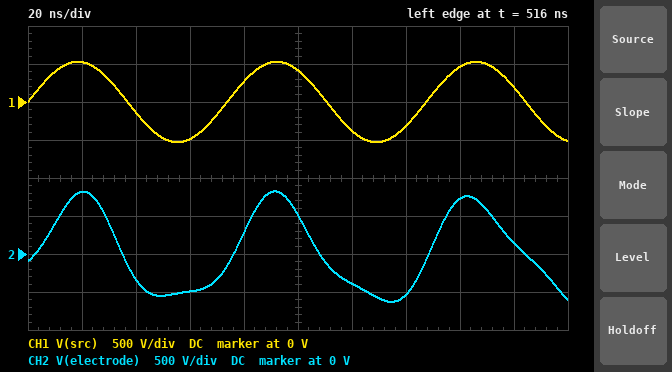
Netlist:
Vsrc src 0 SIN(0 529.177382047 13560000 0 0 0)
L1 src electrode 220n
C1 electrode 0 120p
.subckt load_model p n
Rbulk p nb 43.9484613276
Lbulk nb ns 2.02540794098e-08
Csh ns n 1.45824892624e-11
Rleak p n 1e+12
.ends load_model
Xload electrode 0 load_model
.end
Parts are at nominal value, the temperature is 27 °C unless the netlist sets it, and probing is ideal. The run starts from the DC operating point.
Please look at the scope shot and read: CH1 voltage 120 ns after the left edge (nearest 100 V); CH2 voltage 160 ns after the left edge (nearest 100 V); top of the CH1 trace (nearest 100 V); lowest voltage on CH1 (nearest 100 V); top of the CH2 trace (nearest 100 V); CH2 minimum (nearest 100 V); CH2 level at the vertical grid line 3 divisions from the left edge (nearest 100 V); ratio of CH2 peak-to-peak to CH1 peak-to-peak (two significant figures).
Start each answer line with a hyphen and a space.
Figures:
- -400 V
- 700 V
- 500 V
- -500 V
- 800 V
- -600 V
- -500 V
- 1.4
